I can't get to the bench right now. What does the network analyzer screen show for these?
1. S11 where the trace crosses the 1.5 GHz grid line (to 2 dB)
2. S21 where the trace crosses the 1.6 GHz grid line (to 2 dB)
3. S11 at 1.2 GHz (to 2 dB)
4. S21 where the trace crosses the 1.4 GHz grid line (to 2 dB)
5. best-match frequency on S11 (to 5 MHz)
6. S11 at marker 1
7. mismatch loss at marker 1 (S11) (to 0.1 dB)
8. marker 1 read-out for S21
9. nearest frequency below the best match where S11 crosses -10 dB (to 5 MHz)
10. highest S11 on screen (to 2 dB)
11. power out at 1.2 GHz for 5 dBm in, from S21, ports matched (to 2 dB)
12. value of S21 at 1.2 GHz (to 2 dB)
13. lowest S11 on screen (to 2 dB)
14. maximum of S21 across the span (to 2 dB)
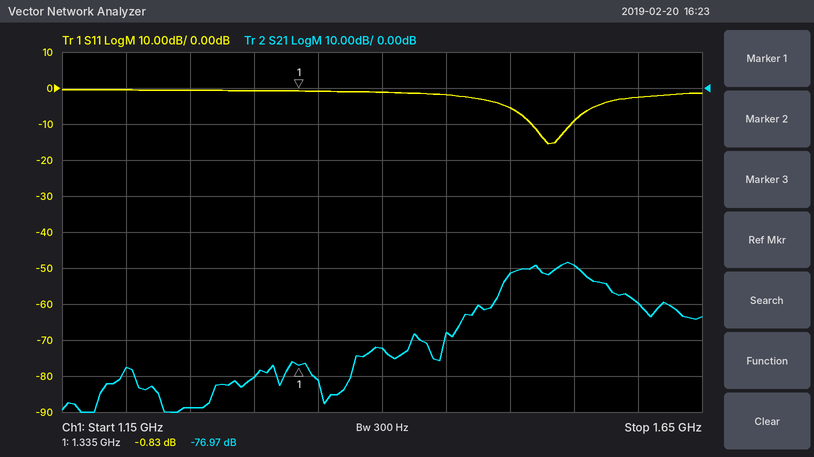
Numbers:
-6 dB
-60 dB
0 dB
-72 dB
1.530 GHz
-0.83 dB
7.6 dB
-76.97 dB
1.515 GHz
0 dB
-72 dBm
-78 dB
-16 dB
-48 dB
